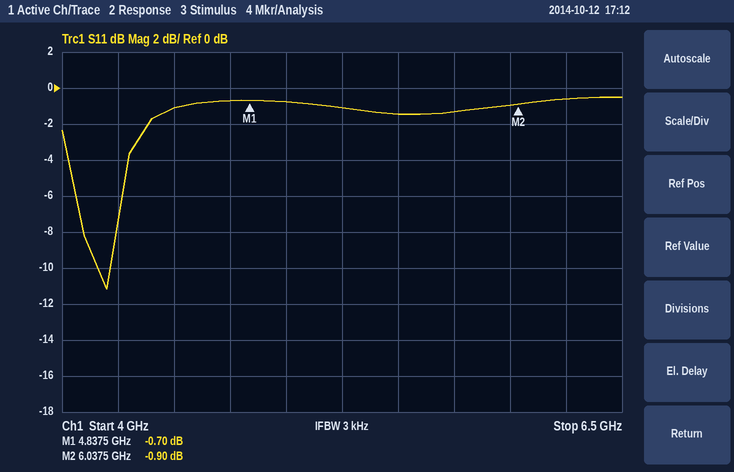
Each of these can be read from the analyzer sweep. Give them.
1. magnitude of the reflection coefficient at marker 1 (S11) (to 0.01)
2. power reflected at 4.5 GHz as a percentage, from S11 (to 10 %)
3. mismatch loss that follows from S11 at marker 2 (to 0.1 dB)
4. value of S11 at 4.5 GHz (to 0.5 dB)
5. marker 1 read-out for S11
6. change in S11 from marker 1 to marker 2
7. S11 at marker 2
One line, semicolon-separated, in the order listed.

0.92; 80 %; 7.3 dB; -1.0 dB; -0.70 dB; -0.20 dB; -0.90 dB
